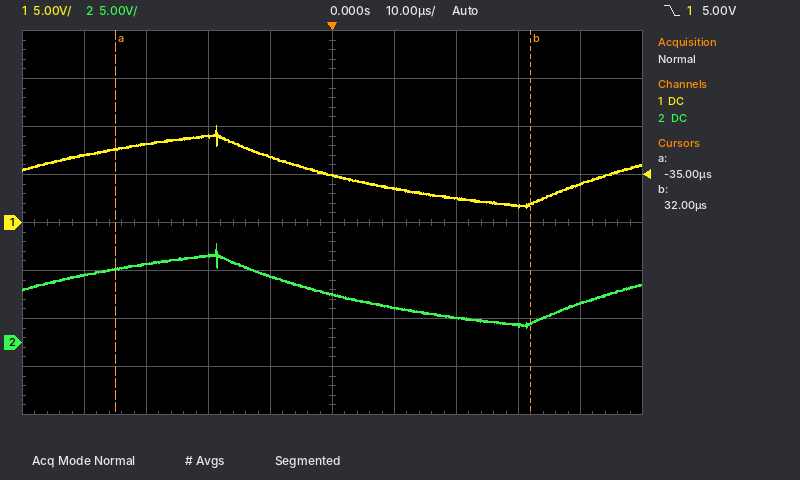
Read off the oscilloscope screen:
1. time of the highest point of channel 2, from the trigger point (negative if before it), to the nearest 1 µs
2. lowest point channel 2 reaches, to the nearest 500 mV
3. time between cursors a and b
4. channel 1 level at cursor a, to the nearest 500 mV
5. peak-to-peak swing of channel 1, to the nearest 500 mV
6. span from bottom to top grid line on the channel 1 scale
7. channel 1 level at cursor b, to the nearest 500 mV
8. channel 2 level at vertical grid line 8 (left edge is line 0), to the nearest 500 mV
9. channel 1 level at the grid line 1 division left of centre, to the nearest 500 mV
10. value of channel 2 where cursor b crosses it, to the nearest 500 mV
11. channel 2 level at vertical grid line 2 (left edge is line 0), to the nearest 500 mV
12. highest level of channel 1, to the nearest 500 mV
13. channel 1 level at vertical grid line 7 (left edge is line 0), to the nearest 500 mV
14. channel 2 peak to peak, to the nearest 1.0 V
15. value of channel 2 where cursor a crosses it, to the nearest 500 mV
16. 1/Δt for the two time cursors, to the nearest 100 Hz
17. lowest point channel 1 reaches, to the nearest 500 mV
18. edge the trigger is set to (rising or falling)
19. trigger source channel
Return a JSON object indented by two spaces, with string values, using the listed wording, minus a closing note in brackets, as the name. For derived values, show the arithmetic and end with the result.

{
  "time of the highest point of channel 2, from the trigger point (negative if before it), to the nearest 1 µs": "-19 µs",
  "lowest point channel 2 reaches, to the nearest 500 mV": "1.5 V",
  "time between cursors a and b": "32 µs − (-35 µs) = 67 µs",
  "channel 1 level at cursor a, to the nearest 500 mV": "7.5 V",
  "peak-to-peak swing of channel 1, to the nearest 500 mV": "10.0 V − (1.5 V) = 8.5 V",
  "span from bottom to top grid line on the channel 1 scale": "40 V",
  "channel 1 level at cursor b, to the nearest 500 mV": "2.0 V",
  "channel 2 level at vertical grid line 8 (left edge is line 0), to the nearest 500 mV": "2.0 V",
  "channel 1 level at the grid line 1 division left of centre, to the nearest 500 mV": "7.0 V",
  "value of channel 2 where cursor b crosses it, to the nearest 500 mV": "2.0 V",
  "channel 2 level at vertical grid line 2 (left edge is line 0), to the nearest 500 mV": "8.0 V",
  "highest level of channel 1, to the nearest 500 mV": "10.0 V",
  "channel 1 level at vertical grid line 7 (left edge is line 0), to the nearest 500 mV": "2.5 V",
  "channel 2 peak to peak, to the nearest 1.0 V": "9.0 V",
  "value of channel 2 where cursor a crosses it, to the nearest 500 mV": "7.5 V",
  "1/Δt for the two time cursors, to the nearest 100 Hz": "1 / 67 µs ≈ 14.9 kHz",
  "lowest point channel 1 reaches, to the nearest 500 mV": "1.5 V",
  "edge the trigger is set to": "falling",
  "trigger source channel": "channel 1"
}
